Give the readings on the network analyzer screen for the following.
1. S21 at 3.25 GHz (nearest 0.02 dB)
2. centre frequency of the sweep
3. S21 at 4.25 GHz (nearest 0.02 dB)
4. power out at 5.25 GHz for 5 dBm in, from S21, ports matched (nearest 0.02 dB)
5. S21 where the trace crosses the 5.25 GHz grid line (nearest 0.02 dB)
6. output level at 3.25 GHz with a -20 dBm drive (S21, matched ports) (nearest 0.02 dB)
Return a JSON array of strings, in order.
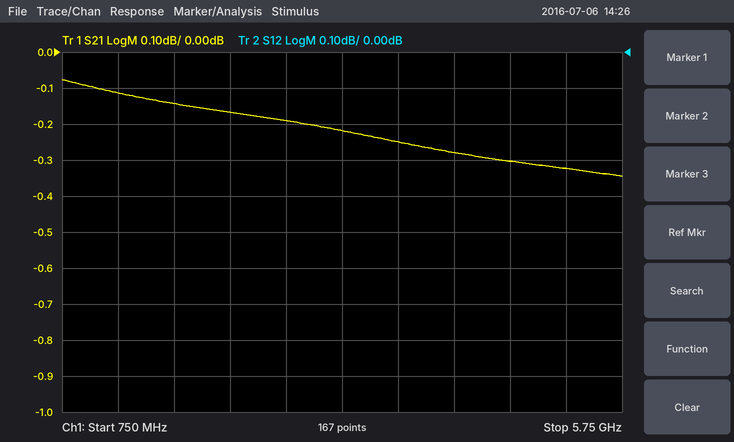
["-0.22 dB", "3.25 GHz", "-0.28 dB", "4.68 dBm", "-0.32 dB", "-20.22 dBm"]
